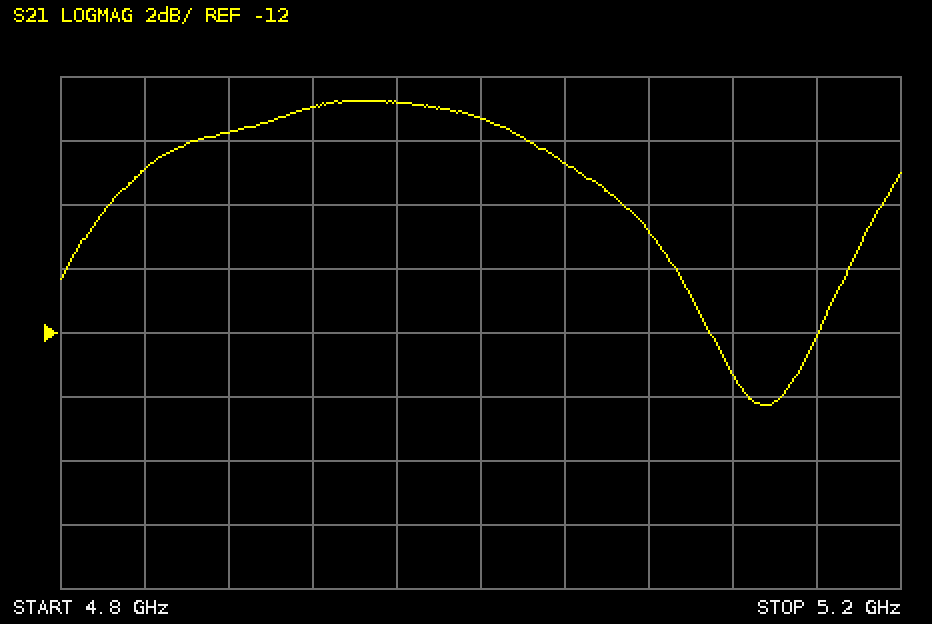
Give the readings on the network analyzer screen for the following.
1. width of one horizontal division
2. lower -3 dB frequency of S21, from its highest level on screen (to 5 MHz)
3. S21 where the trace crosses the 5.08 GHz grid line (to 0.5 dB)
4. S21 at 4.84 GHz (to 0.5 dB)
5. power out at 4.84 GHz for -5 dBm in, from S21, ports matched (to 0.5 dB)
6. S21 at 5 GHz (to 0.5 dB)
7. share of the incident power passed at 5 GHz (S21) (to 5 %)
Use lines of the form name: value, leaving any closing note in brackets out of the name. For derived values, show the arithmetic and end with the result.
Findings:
width of one horizontal division: 40 MHz
lower -3 dB frequency of S21, from its highest level on screen: 4.825 GHz
S21 where the trace crosses the 5.08 GHz grid line: -9.0 dB
S21 at 4.84 GHz: -7.0 dB
power out at 4.84 GHz for -5 dBm in, from S21, ports matched: -5 dBm + (-7.0 dB) = -12.0 dBm
S21 at 5 GHz: -5.5 dB
share of the incident power passed at 5 GHz (S21): 10^(-5.5/10) ≈ 28.2 %, so 30 % to the nearest 5 %
